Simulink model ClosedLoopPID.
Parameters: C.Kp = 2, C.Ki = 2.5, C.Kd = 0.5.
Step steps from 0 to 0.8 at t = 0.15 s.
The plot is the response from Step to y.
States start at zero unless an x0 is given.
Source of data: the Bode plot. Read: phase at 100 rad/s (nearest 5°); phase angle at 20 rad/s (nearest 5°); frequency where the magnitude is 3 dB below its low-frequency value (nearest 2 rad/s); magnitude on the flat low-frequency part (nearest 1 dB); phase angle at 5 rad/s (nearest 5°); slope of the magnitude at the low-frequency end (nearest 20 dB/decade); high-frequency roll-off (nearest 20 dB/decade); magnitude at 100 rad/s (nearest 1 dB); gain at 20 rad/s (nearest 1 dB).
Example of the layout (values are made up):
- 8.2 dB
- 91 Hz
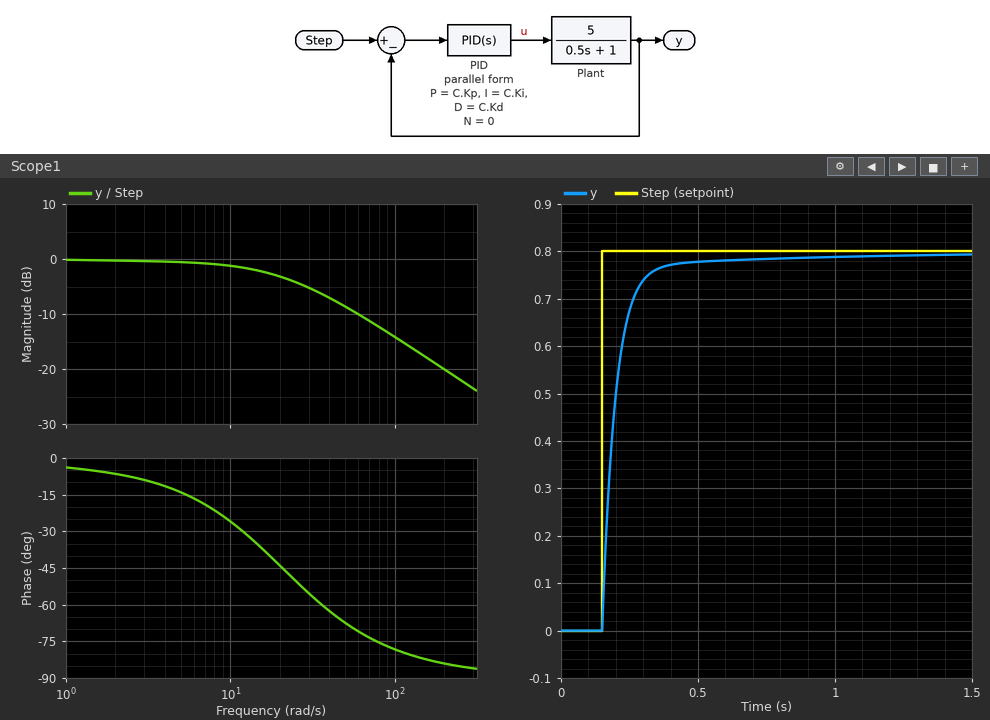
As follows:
- -80°
- -45°
- 20 rad/s
- 0 dB
- -15°
- 0 dB/decade
- -20 dB/decade
- -14 dB
- -3 dB
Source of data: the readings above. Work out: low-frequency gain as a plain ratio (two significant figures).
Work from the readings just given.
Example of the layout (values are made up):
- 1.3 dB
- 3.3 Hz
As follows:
- 1.0
